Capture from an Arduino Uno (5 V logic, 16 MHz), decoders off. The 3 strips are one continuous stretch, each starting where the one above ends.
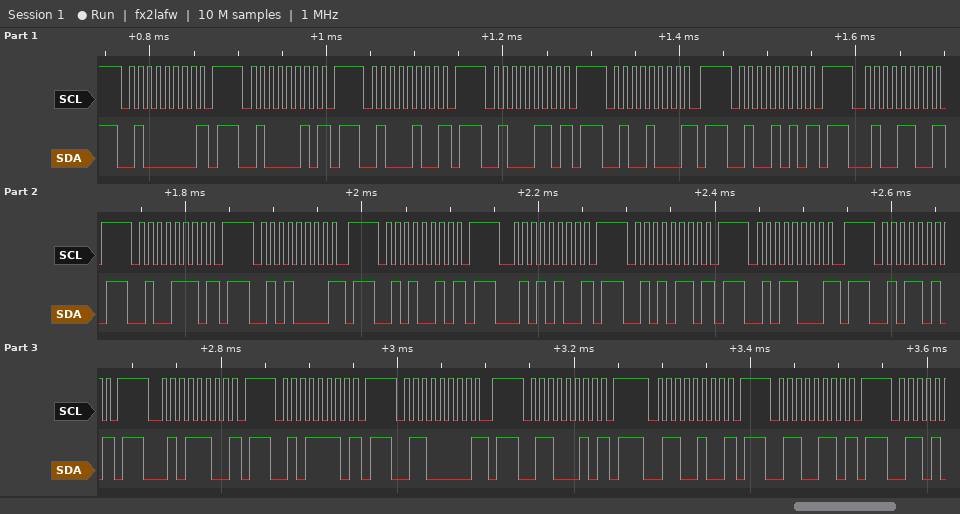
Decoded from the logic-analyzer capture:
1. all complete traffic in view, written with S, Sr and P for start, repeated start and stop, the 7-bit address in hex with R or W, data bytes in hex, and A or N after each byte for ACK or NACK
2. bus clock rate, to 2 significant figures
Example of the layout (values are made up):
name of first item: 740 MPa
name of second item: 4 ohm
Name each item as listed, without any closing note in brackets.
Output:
all complete traffic in view, written with S, Sr and P for start, repeated start and stop, the 7-bit address in hex with R or W, data bytes in hex, and A or N after each byte for ACK or NACK: S 20W N P S 21W N P S 22W N P S 23W N P S 24W N P S 25W N P S 26W N P S 27W N P S 28W N P S 29W N P S 2AW N P S 2BW N P S 2CW N P S 2DW N P S 2EW N P S 2FW N P S 30W N P S 31W N P S 32W N P S 33W N P
bus clock rate, to 2 significant figures: 100 kHz
